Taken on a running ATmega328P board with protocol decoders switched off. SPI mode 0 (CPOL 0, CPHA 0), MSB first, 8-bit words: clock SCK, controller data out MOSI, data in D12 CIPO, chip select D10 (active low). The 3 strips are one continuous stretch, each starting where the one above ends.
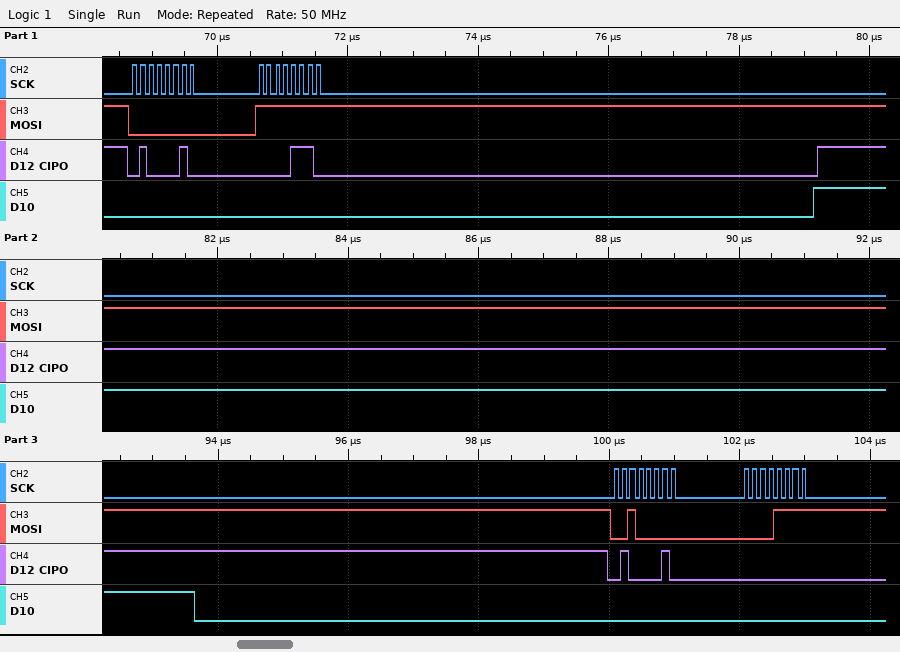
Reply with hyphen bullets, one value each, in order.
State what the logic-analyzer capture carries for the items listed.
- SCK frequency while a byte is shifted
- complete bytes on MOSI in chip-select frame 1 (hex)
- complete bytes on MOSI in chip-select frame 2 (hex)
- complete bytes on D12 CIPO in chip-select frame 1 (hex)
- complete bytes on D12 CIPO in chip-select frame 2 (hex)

- 8 MHz
- 00 FF
- 20 0F
- 42 0E
- 42 00
